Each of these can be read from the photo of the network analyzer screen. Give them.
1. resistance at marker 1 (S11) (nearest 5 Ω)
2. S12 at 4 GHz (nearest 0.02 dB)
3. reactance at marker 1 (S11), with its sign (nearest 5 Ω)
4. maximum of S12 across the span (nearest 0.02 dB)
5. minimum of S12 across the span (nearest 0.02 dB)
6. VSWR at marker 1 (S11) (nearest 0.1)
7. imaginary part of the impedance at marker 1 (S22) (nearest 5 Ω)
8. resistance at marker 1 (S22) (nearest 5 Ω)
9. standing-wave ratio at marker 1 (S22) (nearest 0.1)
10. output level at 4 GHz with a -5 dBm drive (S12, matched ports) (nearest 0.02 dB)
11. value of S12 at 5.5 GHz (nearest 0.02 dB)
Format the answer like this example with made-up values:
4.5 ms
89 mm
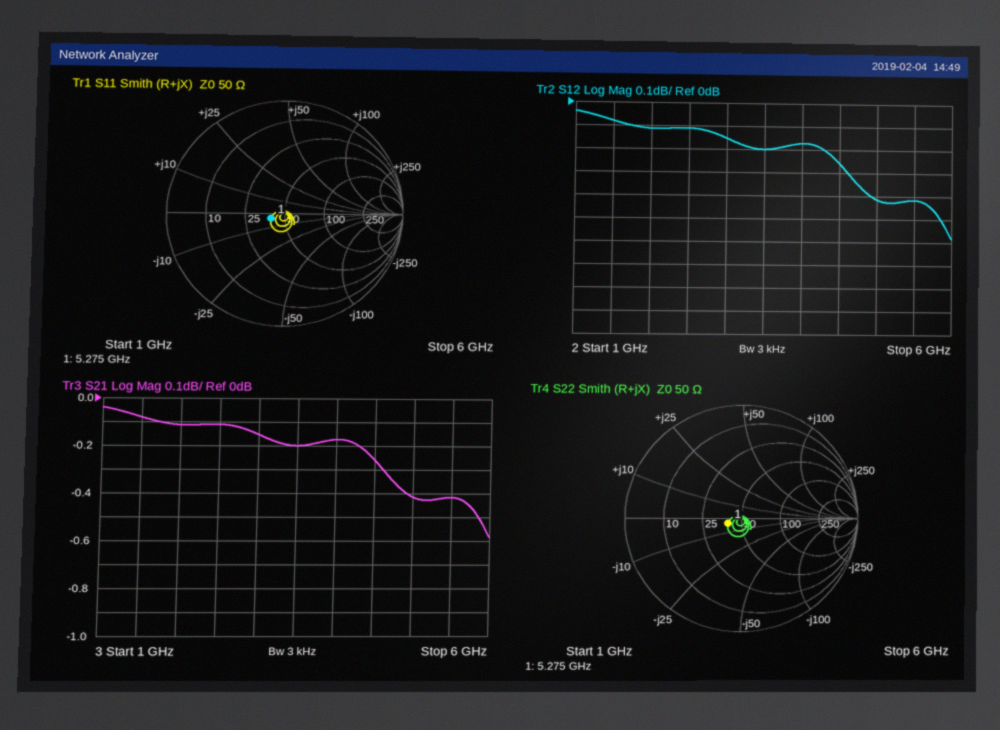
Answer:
40 Ω
-0.18 dB
-5 Ω
-0.04 dB
-0.58 dB
1.3
-5 Ω
40 Ω
1.3
-5.18 dBm
-0.42 dB
